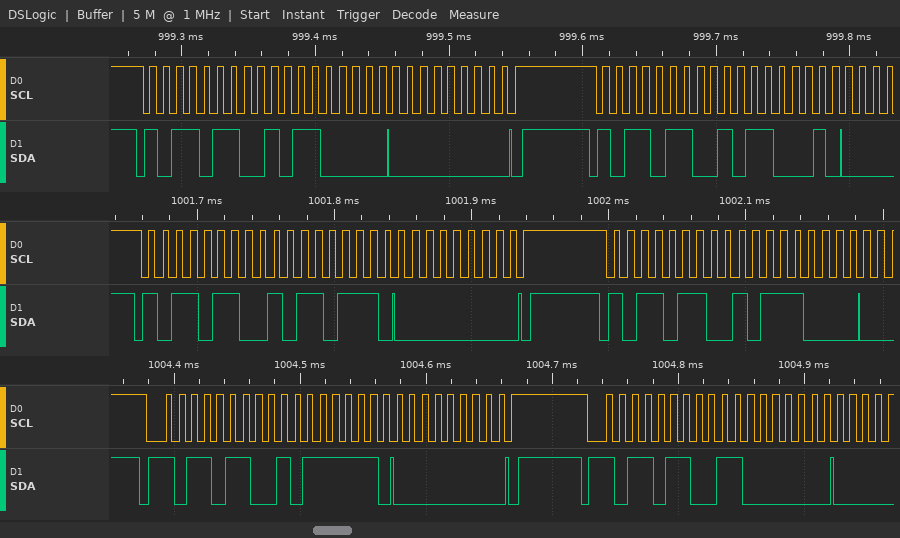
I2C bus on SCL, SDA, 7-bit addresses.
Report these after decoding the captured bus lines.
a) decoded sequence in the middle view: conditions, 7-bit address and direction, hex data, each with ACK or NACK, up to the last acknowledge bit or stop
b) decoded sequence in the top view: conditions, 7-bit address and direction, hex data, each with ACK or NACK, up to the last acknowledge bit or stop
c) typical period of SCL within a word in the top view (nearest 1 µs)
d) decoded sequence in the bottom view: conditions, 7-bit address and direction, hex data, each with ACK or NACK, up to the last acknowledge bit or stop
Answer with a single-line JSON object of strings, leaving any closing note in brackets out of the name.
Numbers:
{"decoded sequence in the middle view: conditions, 7-bit address and direction, hex data, each with ACK or NACK, up to the last acknowledge bit or stop": "start, address 5B write ACK, B7 ACK, 00 ACK, stop, start, address 5B write ACK, B8 ACK", "decoded sequence in the top view: conditions, 7-bit address and direction, hex data, each with ACK or NACK, up to the last acknowledge bit or stop": "start, address 5B write ACK, B0 ACK, 00 ACK, stop, start, address 5B write ACK, B1 ACK", "typical period of SCL within a word in the top view": "10 µs", "decoded sequence in the bottom view: conditions, 7-bit address and direction, hex data, each with ACK or NACK, up to the last acknowledge bit or stop": "start, address 5B write ACK, BF ACK, 00 ACK, stop, start, address 5B write ACK, C0 ACK"}
